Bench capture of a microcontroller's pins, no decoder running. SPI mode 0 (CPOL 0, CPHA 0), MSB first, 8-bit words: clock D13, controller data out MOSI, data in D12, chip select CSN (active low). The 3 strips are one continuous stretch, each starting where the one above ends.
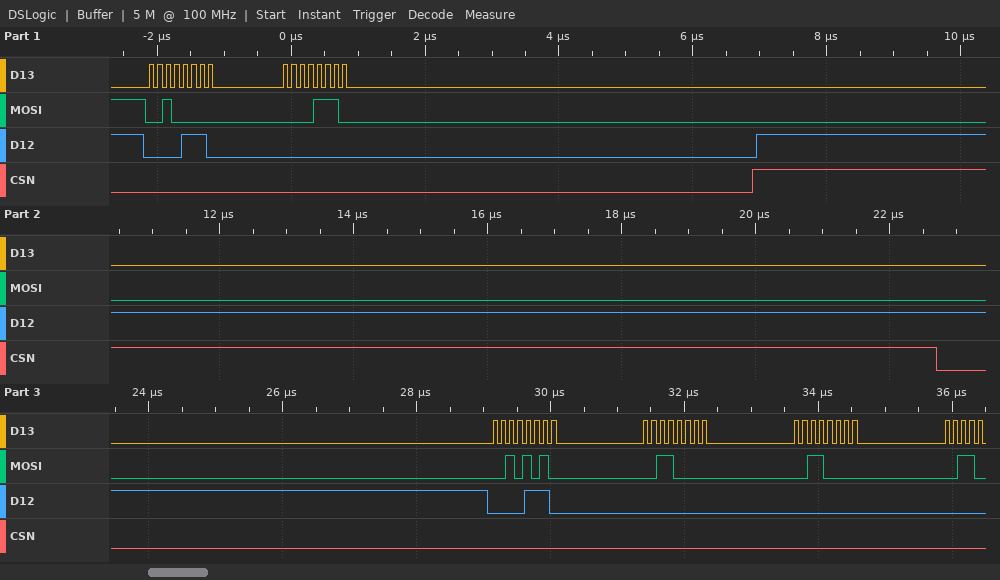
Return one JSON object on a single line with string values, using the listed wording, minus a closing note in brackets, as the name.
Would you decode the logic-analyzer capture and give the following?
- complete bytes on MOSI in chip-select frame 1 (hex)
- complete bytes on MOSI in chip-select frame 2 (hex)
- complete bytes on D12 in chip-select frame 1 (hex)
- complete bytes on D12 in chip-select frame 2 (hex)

{"complete bytes on MOSI in chip-select frame 1": "20 0E", "complete bytes on MOSI in chip-select frame 2": "2A 30 30", "complete bytes on D12 in chip-select frame 1": "0E 00", "complete bytes on D12 in chip-select frame 2": "0E 00 00"}
